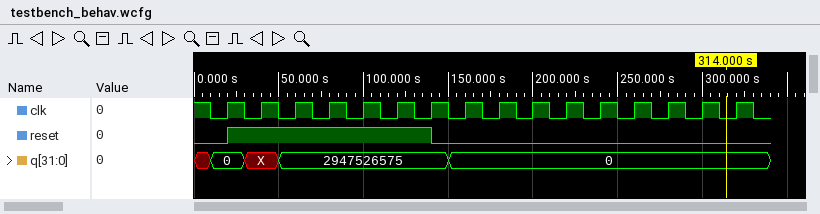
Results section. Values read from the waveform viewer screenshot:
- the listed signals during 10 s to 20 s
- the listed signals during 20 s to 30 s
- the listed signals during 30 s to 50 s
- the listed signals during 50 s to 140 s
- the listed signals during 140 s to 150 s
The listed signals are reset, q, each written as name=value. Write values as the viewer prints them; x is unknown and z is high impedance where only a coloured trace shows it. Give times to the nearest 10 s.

reset=0, q=0
reset=1, q=0
reset=1, q=X
reset=1, q=2947526575
reset=0, q=2947526575
